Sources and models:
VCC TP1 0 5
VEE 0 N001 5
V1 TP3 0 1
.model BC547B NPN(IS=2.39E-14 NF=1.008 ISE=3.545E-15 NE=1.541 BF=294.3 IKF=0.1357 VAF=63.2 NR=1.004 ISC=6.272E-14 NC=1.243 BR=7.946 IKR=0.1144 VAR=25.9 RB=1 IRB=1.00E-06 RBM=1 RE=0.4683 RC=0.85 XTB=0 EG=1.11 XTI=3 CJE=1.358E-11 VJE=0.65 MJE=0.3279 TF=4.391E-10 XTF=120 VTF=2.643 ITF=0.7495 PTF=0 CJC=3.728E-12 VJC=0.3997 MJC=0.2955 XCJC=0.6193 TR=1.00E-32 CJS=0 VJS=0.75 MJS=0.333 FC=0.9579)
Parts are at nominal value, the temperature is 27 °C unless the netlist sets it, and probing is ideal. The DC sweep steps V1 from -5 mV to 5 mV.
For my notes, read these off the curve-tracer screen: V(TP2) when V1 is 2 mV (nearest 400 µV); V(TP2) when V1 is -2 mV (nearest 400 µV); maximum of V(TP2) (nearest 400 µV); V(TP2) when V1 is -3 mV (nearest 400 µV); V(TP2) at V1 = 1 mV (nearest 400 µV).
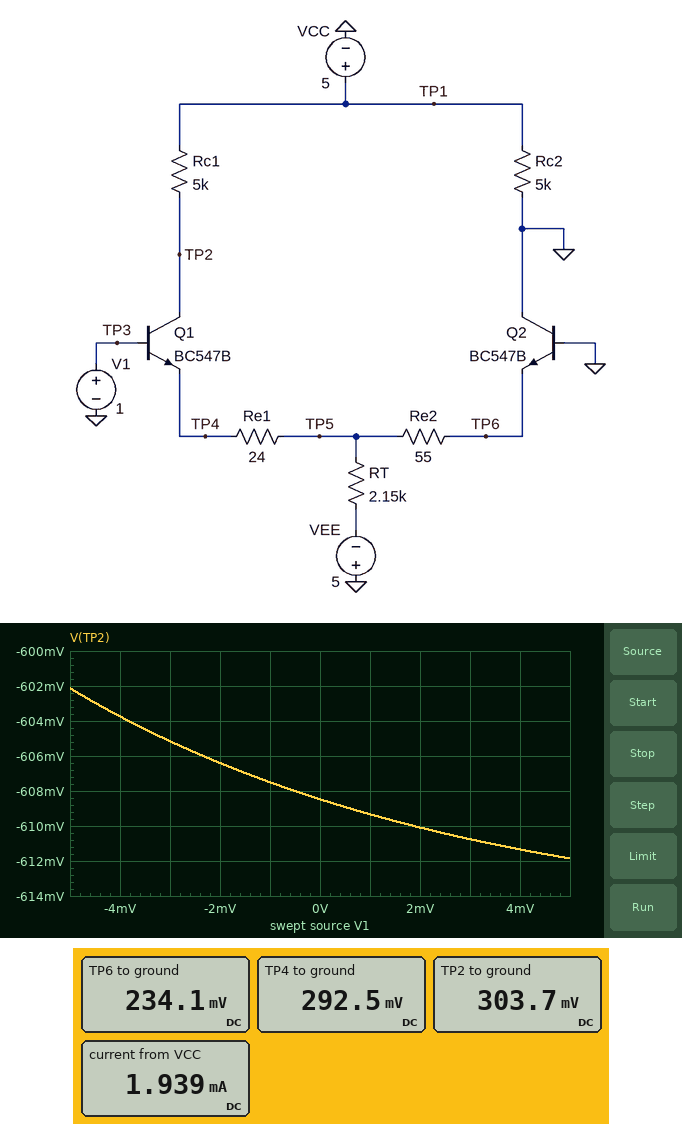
-610.0 mV
-606.4 mV
-602.0 mV
-605.2 mV
-609.2 mV
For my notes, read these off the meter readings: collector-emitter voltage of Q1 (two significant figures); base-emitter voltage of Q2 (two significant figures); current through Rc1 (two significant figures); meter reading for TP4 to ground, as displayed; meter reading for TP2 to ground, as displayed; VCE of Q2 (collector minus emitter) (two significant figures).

11 mV
-230 mV
940 µA
292.5 mV
303.7 mV
-230 mV
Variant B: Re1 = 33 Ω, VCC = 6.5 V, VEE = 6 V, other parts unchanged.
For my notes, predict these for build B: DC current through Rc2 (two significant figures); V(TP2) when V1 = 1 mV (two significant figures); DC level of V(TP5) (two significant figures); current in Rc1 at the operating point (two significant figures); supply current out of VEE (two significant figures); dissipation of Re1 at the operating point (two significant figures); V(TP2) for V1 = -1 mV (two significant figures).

1.3 mA
-570 mV
190 mV
1.2 mA
2.9 mA
270 µW
-550 mV
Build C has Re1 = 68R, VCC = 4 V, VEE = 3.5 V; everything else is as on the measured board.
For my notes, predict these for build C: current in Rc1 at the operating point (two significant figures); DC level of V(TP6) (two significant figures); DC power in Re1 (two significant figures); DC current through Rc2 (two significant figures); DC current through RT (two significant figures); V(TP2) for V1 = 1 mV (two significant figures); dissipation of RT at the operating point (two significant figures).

740 µA
190 mV
200 µW
800 µA
1.7 mA
890 mV
6.3 mW
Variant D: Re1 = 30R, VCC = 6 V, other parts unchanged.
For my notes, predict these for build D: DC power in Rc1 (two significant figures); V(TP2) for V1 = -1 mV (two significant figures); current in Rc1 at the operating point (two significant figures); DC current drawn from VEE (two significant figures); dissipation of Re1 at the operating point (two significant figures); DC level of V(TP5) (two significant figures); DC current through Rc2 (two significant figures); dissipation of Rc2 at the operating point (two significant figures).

6.5 mW
130 mV
1.1 mA
2.4 mA
180 µW
220 mV
1.2 mA
7.2 mW
